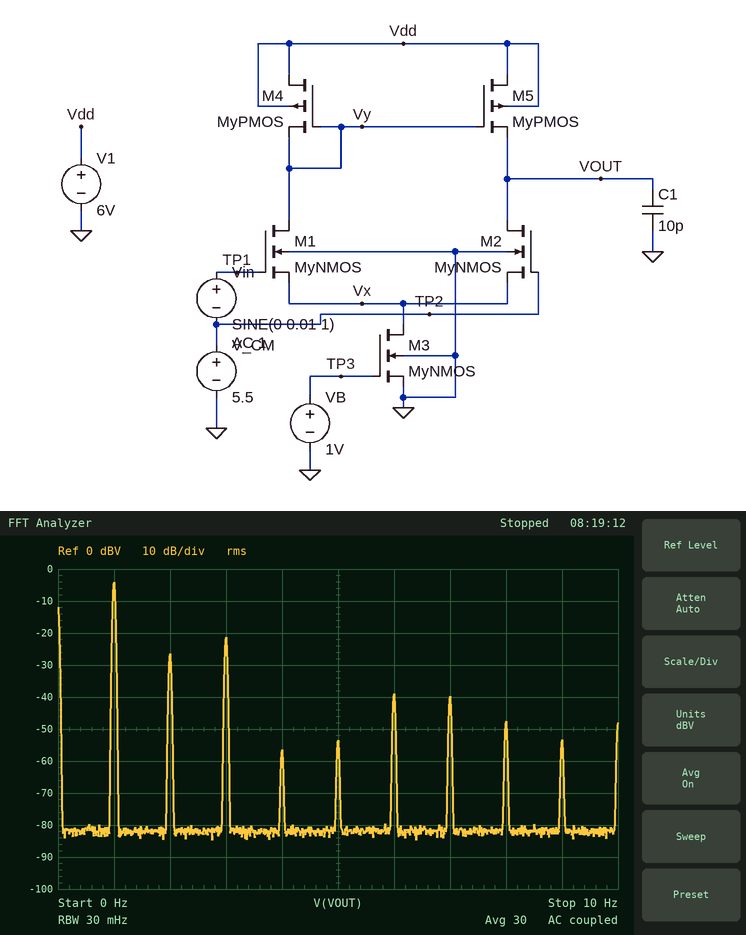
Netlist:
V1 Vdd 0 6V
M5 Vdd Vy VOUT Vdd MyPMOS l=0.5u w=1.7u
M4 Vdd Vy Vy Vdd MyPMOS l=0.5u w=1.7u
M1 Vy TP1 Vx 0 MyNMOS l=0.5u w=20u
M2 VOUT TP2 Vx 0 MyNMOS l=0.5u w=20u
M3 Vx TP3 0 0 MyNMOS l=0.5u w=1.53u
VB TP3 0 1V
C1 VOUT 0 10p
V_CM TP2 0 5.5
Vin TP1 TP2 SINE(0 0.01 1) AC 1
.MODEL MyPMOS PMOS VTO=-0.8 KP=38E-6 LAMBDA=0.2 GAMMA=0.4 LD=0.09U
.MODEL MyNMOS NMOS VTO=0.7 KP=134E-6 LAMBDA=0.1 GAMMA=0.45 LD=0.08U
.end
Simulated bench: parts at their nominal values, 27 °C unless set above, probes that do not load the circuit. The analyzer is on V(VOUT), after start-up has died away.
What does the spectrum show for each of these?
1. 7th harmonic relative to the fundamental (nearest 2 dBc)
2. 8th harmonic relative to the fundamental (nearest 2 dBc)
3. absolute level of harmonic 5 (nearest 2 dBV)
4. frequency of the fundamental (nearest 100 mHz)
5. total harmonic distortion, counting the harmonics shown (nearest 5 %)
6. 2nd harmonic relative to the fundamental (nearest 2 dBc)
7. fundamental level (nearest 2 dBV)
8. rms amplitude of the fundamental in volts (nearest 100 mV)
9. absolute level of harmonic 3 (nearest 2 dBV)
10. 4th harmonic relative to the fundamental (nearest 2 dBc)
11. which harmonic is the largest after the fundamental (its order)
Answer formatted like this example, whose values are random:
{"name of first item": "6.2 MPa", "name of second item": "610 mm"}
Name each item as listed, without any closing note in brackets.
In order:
{"7th harmonic relative to the fundamental": "-36 dBc", "8th harmonic relative to the fundamental": "-44 dBc", "absolute level of harmonic 5": "-54 dBV", "frequency of the fundamental": "1.0 Hz", "total harmonic distortion, counting the harmonics shown": "15 %", "2nd harmonic relative to the fundamental": "-22 dBc", "fundamental level": "-4 dBV", "rms amplitude of the fundamental in volts": "600 mV", "absolute level of harmonic 3": "-22 dBV", "4th harmonic relative to the fundamental": "-52 dBc", "which harmonic is the largest after the fundamental": "3"}
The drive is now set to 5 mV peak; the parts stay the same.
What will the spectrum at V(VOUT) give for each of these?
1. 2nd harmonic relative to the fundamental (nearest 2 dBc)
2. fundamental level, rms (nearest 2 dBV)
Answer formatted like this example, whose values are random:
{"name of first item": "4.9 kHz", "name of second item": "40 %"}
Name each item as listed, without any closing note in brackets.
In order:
{"2nd harmonic relative to the fundamental": "-50 dBc", "fundamental level, rms": "-8 dBV"}
